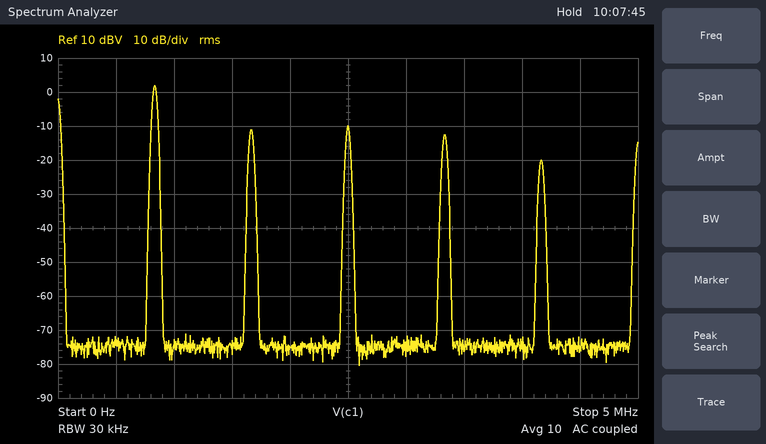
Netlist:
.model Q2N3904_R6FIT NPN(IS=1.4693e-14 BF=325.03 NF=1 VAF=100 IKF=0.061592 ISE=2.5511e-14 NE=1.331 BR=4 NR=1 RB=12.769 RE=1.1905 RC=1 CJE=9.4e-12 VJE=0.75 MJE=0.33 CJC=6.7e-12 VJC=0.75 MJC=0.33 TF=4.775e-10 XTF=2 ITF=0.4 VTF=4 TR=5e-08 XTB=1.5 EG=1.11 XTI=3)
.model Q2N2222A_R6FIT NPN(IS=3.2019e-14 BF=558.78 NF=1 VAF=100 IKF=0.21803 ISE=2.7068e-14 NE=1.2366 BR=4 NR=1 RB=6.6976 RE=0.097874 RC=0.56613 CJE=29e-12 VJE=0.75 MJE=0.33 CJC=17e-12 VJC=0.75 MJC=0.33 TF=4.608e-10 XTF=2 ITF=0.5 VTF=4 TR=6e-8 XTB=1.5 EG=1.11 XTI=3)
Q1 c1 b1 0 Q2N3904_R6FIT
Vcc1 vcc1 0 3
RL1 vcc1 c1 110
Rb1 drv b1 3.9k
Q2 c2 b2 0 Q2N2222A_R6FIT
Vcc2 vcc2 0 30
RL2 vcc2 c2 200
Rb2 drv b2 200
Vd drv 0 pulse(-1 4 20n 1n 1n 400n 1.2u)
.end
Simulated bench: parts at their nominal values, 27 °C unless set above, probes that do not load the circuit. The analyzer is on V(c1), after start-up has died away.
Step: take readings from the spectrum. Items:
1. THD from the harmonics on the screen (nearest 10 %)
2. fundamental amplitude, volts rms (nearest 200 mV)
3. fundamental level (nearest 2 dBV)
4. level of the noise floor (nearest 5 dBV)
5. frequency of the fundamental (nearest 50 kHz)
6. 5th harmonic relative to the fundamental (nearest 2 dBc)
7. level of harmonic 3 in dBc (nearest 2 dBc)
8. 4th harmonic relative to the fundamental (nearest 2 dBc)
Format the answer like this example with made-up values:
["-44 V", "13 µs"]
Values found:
["40 %", "1.2 V", "2 dBV", "-75 dBV", "850 kHz", "-22 dBc", "-12 dBc", "-14 dBc"]
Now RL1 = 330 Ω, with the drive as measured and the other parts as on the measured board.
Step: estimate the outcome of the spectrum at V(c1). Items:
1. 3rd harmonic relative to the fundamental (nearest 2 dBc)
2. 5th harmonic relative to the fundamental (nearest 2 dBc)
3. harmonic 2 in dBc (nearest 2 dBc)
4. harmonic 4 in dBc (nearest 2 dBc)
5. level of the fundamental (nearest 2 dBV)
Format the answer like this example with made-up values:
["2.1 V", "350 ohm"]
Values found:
["-10 dBc", "-16 dBc", "-20 dBc", "-20 dBc", "2 dBV"]
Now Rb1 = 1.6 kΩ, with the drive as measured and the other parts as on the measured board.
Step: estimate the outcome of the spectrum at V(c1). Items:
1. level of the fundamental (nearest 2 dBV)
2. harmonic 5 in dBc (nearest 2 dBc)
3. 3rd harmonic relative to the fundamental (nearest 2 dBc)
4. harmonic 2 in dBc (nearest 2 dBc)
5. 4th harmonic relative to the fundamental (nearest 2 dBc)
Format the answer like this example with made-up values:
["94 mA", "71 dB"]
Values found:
["2 dBV", "-16 dBc", "-10 dBc", "-18 dBc", "-20 dBc"]
